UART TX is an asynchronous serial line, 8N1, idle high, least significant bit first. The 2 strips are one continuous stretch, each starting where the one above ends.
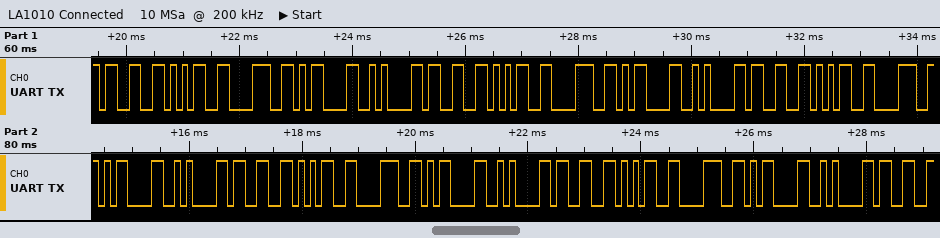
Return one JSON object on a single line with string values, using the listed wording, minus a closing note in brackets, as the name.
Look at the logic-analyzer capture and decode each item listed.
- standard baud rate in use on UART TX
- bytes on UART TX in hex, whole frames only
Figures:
{"standard baud rate in use on UART TX": "9600 baud", "bytes on UART TX in hex, whole frames only": "33 35 38 0D 0A 33 35 38 0D 0A 33 35 38 0D 0A 33 35 38 0D 0A 33 35 38 0D 0A 33"}
